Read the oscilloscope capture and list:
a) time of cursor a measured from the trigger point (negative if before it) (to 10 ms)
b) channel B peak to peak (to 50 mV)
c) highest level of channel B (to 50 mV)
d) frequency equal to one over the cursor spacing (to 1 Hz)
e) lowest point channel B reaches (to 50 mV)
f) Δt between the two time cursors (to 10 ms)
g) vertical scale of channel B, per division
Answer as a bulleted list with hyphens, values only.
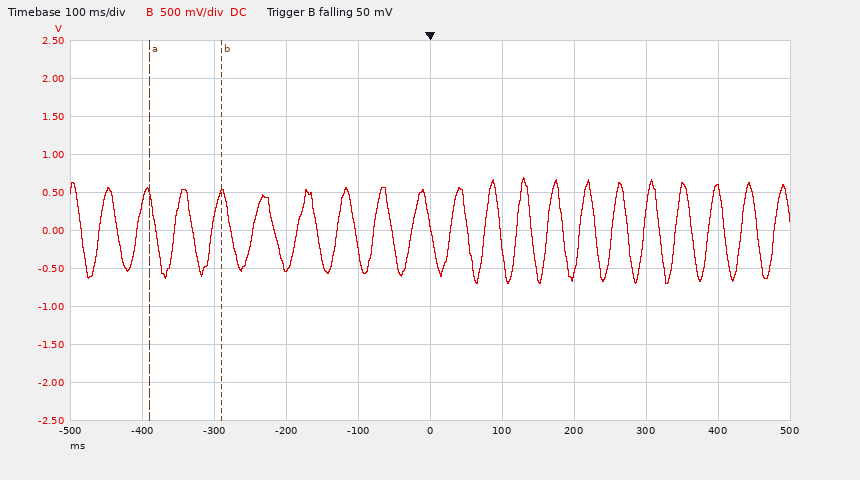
- -390 ms
- 1.40 V
- 700 mV
- 10 Hz
- -700 mV
- 100 ms
- 500 mV
